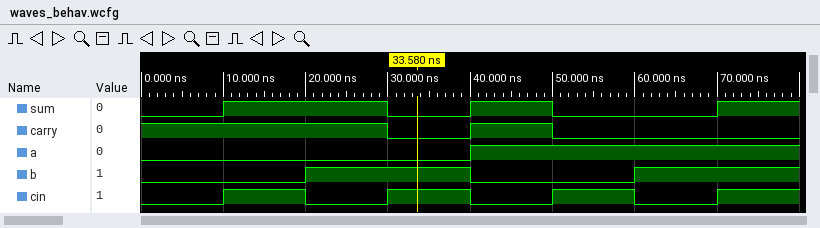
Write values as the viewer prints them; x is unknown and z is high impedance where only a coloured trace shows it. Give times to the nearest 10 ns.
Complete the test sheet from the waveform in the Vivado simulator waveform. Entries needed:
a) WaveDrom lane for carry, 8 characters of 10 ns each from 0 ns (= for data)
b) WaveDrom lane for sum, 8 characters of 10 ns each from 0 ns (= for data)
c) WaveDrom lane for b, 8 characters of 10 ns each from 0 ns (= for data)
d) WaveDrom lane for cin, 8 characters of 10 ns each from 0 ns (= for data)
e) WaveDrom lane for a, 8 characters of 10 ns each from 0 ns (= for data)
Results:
{name: 'carry', wave: '1..010..'}
{name: 'sum', wave: '01.010.1'}
{name: 'b', wave: '0.1.0.1.'}
{name: 'cin', wave: '01010101'}
{name: 'a', wave: '0...1...'}
